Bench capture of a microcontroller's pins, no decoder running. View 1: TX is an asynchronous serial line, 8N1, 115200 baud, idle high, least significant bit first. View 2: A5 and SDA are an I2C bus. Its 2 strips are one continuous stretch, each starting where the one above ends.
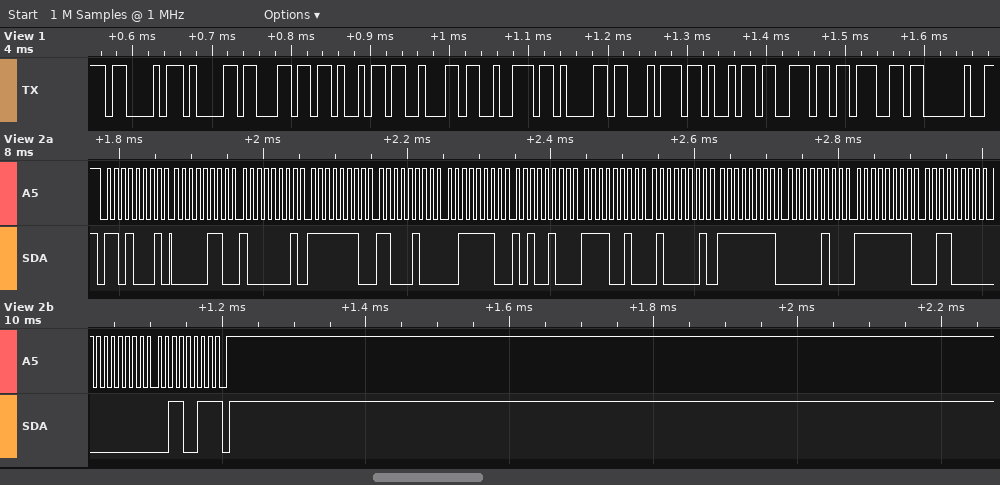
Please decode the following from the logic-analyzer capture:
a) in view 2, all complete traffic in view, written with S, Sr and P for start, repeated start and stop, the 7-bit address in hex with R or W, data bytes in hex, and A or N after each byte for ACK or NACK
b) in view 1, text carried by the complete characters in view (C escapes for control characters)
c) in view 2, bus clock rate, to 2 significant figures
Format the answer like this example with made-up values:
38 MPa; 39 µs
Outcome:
S 68R A 06 A 81 A FE A C4 A 3E A A4 A F2 A 41 A FF A 04 A FF A 30 A 00 A 33 N P; "Calibrating "; 100 kHz
